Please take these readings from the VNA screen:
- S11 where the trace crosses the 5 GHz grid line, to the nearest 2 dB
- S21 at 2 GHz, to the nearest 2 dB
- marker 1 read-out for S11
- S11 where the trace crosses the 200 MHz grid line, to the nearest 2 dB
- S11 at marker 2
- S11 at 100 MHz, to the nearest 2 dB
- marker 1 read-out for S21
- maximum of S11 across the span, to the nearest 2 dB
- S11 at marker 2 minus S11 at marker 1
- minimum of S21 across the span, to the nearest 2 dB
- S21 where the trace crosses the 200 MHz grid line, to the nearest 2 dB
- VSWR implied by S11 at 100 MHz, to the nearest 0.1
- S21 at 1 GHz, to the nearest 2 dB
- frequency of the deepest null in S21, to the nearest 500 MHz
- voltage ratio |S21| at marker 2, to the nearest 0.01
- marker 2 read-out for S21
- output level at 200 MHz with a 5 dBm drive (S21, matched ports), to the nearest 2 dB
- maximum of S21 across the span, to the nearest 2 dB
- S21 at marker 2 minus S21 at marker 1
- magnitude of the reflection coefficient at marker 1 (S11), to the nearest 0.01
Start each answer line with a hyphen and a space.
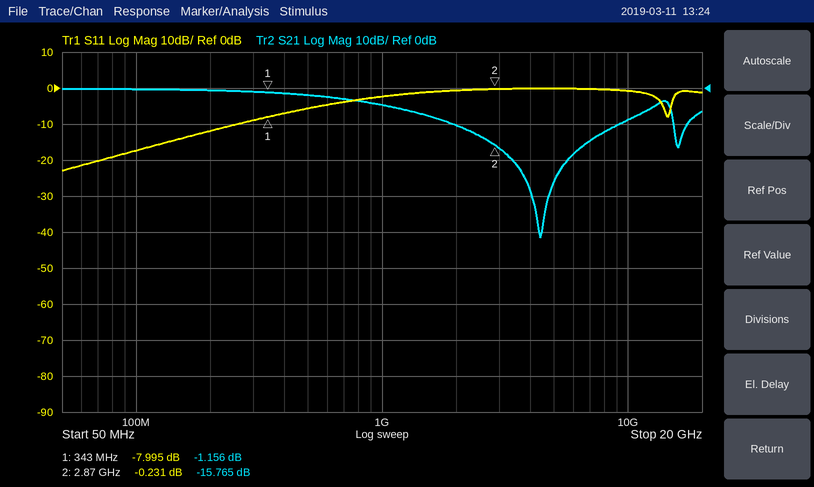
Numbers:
- 0 dB
- -10 dB
- -7.995 dB
- -12 dB
- -0.231 dB
- -18 dB
- -1.156 dB
- 0 dB
- 7.764 dB
- -42 dB
- 0 dB
- 1.3
- -4 dB
- 4.5 GHz
- 0.16
- -15.765 dB
- 4 dBm
- 0 dB
- -14.609 dB
- 0.40
